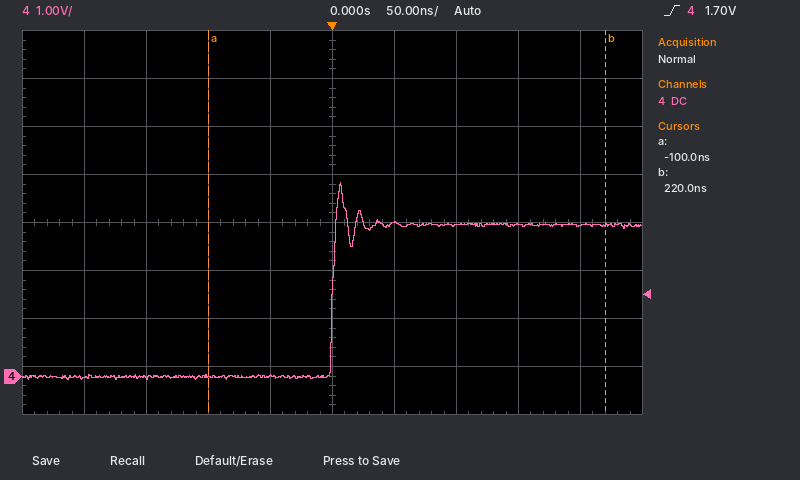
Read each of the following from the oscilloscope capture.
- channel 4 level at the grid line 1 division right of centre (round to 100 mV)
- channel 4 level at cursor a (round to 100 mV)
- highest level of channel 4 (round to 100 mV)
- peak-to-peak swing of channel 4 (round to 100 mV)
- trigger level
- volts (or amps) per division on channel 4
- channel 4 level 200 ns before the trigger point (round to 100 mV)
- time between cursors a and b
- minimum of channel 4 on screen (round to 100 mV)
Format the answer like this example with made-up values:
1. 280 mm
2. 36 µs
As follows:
1. 3.2 V
2. 0.0 V
3. 4.0 V
4. 4.1 V
5. 1.70 V
6. 1 V
7. 0.0 V
8. 320 ns
9. -100 mV
